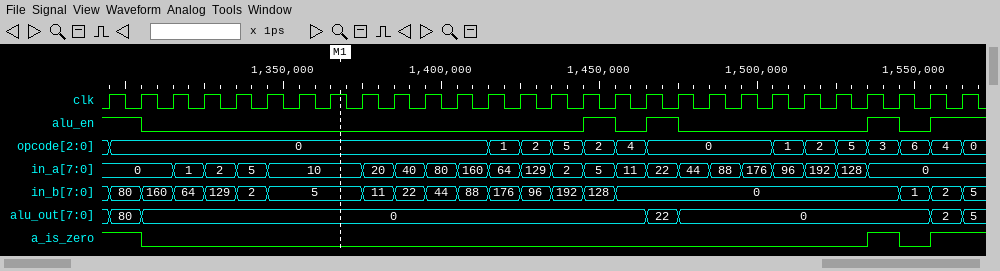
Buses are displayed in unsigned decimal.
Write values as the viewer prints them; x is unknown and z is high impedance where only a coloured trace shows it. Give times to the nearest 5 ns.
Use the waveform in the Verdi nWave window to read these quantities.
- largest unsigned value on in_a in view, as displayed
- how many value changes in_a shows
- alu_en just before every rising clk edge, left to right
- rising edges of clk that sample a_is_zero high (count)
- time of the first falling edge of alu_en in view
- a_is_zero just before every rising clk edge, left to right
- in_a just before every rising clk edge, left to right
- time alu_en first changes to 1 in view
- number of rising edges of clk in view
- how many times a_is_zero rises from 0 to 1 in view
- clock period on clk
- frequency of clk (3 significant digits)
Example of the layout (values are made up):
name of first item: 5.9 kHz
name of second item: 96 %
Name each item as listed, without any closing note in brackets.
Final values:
largest unsigned value on in_a in view, as displayed: 192
how many value changes in_a shows: 21
alu_en just before every rising clk edge, left to right: 1 1 0 0 0 0 0 0 0 0 0 0 0 0 0 0 1 0 1 0 0 0 0 0 0 1 0 1
rising edges of clk that sample a_is_zero high: 4
time of the first falling edge of alu_en in view: 1305 ns
a_is_zero just before every rising clk edge, left to right: 1 1 0 0 0 0 0 0 0 0 0 0 0 0 0 0 0 0 0 0 0 0 0 0 0 1 0 1
in_a just before every rising clk edge, left to right: 0, 0, 0, 1, 2, 5, 10, 10, 10, 20, 40, 80, 160, 64, 129, 2, 5, 11, 22, 44, 88, 176, 96, 192, 128, 0, 0, 0
time alu_en first changes to 1 in view: 1445 ns
number of rising edges of clk in view: 28
how many times a_is_zero rises from 0 to 1 in view: 2
clock period on clk: 10 ns
frequency of clk: 100 MHz
